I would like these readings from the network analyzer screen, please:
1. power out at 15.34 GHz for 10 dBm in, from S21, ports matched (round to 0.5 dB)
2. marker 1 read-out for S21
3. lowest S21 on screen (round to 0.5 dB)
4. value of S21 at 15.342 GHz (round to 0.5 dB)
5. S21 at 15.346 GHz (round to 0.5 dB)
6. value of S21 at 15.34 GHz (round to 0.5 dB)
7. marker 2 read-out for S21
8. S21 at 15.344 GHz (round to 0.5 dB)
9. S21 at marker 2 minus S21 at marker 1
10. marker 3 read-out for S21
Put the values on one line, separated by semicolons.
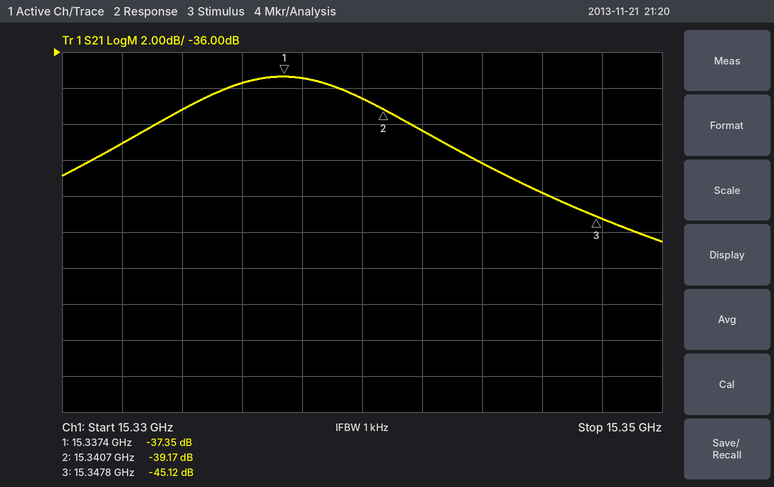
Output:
-28.5 dBm; -37.35 dB; -46.5 dB; -40.5 dB; -44.0 dB; -38.5 dB; -39.17 dB; -42.0 dB; -1.82 dB; -45.12 dB
